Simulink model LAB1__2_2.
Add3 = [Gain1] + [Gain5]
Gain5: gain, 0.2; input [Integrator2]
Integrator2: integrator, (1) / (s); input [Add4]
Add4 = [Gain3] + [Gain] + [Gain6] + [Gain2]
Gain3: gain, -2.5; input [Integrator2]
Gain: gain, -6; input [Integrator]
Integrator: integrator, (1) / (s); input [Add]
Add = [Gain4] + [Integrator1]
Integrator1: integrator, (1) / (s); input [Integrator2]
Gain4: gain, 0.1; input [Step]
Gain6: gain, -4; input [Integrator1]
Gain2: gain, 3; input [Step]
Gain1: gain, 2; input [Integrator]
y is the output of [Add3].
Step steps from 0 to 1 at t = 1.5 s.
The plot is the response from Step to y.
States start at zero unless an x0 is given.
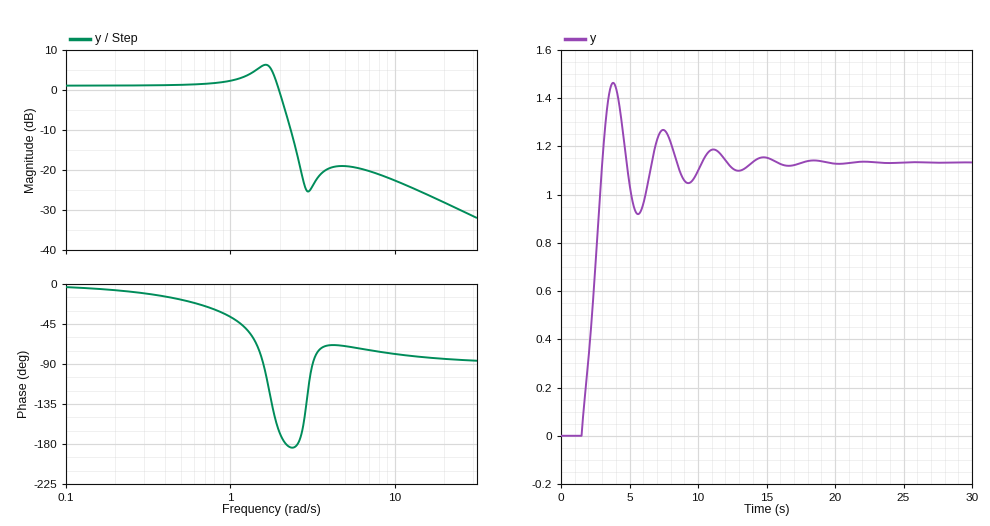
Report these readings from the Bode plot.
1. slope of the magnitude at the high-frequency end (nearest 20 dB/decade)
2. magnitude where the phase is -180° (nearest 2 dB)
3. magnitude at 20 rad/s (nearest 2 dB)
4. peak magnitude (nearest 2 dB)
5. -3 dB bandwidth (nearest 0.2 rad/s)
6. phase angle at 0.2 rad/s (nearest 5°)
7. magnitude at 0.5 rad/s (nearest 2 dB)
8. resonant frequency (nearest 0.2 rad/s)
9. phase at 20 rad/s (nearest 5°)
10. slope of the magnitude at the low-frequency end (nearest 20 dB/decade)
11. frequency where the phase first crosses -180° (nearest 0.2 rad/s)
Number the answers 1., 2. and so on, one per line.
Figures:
1. -20 dB/decade
2. -6 dB
3. -28 dB
4. 6 dB
5. 2.0 rad/s
6. -5°
7. 2 dB
8. 1.6 rad/s
9. -85°
10. 0 dB/decade
11. 2.2 rad/s
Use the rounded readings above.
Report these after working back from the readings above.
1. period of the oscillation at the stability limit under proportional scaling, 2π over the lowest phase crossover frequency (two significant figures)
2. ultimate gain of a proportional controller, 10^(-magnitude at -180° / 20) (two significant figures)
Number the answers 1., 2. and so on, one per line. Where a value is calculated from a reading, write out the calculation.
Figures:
1. 2π / 2.2 = 2.9 s
2. 10^(6 / 20) = 2.0
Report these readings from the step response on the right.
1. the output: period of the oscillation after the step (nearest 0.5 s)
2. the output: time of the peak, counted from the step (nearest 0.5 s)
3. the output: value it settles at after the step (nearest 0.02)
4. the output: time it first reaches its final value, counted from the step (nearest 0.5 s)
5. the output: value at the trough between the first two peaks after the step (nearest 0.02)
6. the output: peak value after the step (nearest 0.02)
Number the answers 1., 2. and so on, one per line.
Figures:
1. 3.5 s
2. 2.5 s
3. 1.14
4. 1.5 s
5. 0.92
6. 1.46
